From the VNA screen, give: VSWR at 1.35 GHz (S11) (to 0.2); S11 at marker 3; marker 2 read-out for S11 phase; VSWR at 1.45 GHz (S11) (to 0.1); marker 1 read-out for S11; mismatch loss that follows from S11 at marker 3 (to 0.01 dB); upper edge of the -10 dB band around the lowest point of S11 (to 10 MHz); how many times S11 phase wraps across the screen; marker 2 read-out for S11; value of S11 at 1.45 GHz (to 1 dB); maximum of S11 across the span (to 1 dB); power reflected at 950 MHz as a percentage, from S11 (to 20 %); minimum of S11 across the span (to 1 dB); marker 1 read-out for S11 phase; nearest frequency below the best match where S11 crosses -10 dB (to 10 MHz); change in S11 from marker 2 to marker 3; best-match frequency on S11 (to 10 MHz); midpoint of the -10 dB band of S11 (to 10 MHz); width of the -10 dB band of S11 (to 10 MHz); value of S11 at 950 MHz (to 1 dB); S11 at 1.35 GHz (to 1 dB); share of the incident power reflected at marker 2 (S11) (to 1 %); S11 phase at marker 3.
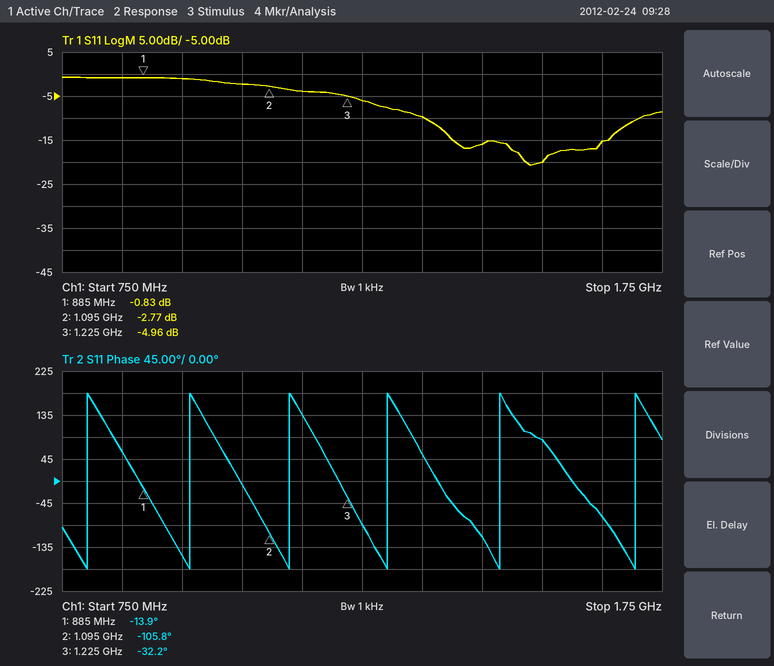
2.0
-4.96 dB
-105.8°
1.4
-0.83 dB
1.67 dB
1.71 GHz
6
-2.77 dB
-16 dB
-1 dB
80 %
-21 dB
-13.9°
1.35 GHz
-2.19 dB
1.53 GHz
1.53 GHz
360 MHz
-1 dB
-10 dB
53 %
-32.2°
